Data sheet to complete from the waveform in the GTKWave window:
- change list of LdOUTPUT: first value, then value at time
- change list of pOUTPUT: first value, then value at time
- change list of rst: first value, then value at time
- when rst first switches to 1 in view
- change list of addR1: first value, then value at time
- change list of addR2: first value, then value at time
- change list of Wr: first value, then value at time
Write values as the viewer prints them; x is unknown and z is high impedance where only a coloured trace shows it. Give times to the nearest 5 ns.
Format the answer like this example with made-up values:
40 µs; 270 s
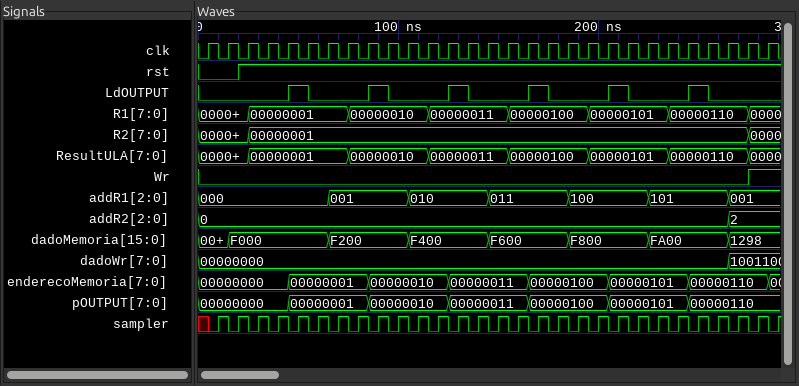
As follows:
0, 1 at 45 ns, 0 at 55 ns, 1 at 85 ns, 0 at 95 ns, 1 at 125 ns, 0 at 135 ns, 1 at 165 ns, 0 at 175 ns, 1 at 205 ns, 0 at 215 ns, 1 at 245 ns, 0 at 255 ns; 00000000, 00000001 at 45 ns, 00000010 at 85 ns, 00000011 at 125 ns, 00000100 at 165 ns, 00000101 at 205 ns, 00000110 at 245 ns; 0, 1 at 20 ns; 20 ns; 000, 001 at 65 ns, 010 at 105 ns, 011 at 145 ns, 100 at 185 ns, 101 at 225 ns, 001 at 265 ns; 0, 2 at 265 ns; 0, 1 at 275 ns
